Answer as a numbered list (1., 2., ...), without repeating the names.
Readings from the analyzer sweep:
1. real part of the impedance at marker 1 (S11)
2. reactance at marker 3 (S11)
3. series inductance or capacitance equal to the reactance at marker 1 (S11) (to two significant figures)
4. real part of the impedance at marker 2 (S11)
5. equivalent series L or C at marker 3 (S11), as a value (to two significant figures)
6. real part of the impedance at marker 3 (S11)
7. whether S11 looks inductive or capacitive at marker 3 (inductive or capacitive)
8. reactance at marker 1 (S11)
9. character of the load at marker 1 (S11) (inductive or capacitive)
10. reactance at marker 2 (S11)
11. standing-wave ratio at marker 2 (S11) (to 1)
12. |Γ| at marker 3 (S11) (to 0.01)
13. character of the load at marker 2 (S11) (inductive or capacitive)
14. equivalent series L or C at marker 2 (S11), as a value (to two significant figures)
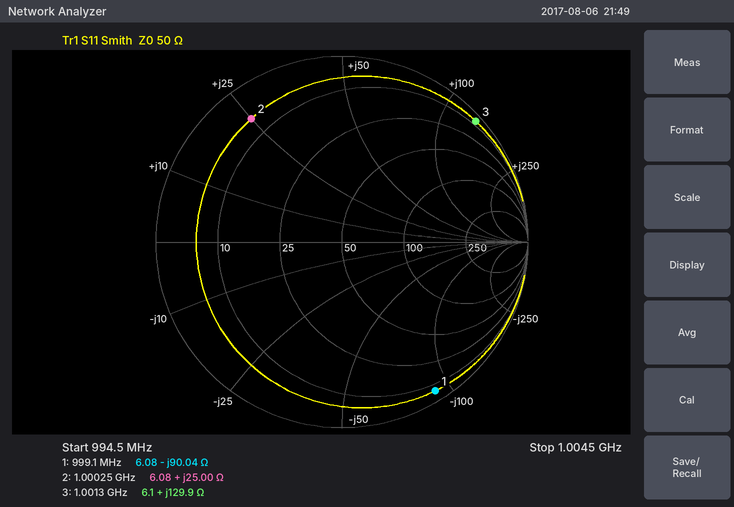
1. 6.08 Ω
2. +129.9 Ω
3. 1.8 pF
4. 6.08 Ω
5. 21 nH
6. 6.1 Ω
7. inductive
8. -90.04 Ω
9. capacitive
10. +25.00 Ω
11. 10
12. 0.97
13. inductive
14. 4.0 nH
